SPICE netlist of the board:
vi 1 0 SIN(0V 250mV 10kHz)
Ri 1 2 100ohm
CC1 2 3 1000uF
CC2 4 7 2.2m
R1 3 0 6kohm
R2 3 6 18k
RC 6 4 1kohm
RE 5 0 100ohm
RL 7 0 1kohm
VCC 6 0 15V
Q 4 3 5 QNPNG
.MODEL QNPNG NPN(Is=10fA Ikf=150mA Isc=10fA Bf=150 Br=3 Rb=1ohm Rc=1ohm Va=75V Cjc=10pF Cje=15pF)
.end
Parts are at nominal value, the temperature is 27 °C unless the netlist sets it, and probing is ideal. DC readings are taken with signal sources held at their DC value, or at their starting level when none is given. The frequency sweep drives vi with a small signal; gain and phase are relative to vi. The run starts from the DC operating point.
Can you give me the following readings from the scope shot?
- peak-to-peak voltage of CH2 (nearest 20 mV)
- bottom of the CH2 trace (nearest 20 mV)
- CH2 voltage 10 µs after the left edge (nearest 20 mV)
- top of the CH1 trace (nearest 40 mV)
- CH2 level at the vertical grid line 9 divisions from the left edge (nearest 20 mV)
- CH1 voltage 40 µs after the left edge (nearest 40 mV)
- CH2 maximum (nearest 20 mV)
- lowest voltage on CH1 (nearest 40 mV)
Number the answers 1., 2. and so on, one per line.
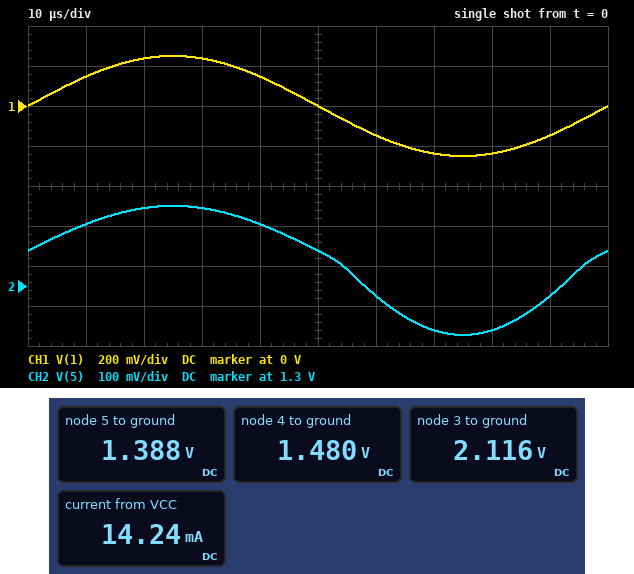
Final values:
1. 320 mV
2. 1.18 V
3. 1.46 V
4. 240 mV
5. 1.28 V
6. 160 mV
7. 1.50 V
8. -240 mV
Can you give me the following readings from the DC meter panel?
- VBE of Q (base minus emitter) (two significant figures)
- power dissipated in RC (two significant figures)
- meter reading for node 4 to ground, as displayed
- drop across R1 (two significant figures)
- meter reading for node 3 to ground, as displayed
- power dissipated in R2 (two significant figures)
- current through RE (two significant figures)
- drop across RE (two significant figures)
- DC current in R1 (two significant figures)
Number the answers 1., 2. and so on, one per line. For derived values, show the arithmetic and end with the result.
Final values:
1. 2.116 V - 1.388 V = 730 mV
2. (15 V - 1.48 V)^2 / 1 kΩ = 180 mW
3. 1.480 V
4. 2.116 V = 2.1 V
5. 2.116 V
6. (15 V - 2.116 V)^2 / 18 kΩ = 9.2 mW
7. (1.388 V) / 100 Ω = 14 mA
8. 1.388 V = 1.4 V
9. (2.116 V) / 6 kΩ = 350 µA
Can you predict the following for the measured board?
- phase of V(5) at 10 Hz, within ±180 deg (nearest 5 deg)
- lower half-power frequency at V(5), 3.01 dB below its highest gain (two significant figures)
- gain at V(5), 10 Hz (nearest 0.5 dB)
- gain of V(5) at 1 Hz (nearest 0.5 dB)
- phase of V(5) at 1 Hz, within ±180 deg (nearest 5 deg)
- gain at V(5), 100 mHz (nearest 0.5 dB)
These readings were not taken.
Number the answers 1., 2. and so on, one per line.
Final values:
1. 5 deg
2. 780 mHz
3. -6.5 dB
4. -8.5 dB
5. 40 deg
6. -24.5 dB
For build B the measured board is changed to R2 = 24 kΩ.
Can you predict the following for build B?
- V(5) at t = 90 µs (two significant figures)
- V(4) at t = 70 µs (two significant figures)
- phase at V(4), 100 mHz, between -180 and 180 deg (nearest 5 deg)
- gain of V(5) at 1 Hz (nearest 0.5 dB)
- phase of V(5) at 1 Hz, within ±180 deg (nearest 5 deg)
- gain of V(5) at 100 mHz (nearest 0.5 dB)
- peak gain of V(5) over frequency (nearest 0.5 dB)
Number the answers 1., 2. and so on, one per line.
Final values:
1. 1.2 V
2. 2.5 V
3. -100 deg
4. -7.0 dB
5. 35 deg
6. -22.5 dB
7. -5.5 dB
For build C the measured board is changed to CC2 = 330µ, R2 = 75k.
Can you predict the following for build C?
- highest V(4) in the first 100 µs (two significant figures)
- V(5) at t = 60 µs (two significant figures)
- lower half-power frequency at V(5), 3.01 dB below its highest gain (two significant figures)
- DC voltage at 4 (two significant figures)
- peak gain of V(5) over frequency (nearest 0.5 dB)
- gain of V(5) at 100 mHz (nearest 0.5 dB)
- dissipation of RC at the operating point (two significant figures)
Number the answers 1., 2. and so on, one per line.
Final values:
1. 13 V
2. 190 mV
3. 37 mHz
4. 12 V
5. -1.0 dB
6. -1.5 dB
7. 10 mW
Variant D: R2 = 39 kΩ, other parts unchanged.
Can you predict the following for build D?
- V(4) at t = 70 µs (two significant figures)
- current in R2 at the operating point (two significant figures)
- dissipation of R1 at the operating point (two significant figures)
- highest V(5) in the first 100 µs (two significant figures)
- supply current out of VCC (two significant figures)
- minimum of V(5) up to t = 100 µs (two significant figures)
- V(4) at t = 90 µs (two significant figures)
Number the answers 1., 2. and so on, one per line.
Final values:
1. 6.6 V
2. 340 µA
3. 460 µW
4. 1.2 V
5. 9.8 mA
6. 720 mV
7. 6.2 V
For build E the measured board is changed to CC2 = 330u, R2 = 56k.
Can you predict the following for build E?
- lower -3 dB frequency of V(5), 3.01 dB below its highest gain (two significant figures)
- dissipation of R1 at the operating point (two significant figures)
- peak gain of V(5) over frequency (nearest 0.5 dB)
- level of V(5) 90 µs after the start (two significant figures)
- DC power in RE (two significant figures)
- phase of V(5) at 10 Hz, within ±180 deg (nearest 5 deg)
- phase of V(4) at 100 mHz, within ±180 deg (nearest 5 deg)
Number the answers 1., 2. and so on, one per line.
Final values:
1. 39 mHz
2. 270 µW
3. -0.5 dB
4. 430 mV
5. 3.2 mW
6. 0 deg
7. -170 deg
